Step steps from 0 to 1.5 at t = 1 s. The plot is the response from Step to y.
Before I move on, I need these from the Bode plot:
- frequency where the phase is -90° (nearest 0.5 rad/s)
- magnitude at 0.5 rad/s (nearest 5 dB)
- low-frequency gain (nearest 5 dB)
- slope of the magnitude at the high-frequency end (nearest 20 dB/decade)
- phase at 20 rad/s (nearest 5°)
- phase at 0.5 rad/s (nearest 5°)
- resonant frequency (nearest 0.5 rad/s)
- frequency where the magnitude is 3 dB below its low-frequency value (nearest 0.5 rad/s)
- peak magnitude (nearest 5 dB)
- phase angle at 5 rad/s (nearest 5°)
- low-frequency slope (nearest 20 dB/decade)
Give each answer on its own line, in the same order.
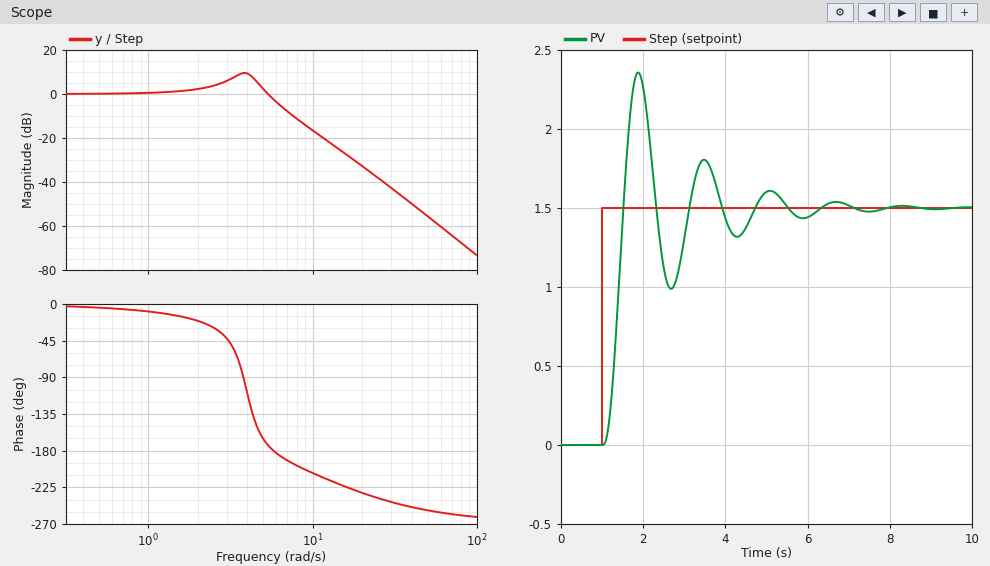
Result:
4.0 rad/s
0 dB
0 dB
-60 dB/decade
-230°
-5°
4.0 rad/s
6.0 rad/s
10 dB
-165°
0 dB/decade
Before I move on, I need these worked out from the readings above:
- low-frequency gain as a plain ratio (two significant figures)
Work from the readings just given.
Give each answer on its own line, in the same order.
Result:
1.0
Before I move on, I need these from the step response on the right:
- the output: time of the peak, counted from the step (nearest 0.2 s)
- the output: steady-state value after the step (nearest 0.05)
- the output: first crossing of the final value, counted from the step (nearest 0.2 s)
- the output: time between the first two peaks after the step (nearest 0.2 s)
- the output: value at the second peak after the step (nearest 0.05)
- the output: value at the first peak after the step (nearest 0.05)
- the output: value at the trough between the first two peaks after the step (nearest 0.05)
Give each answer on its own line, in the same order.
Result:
0.8 s
1.50
0.6 s
1.6 s
1.80
2.35
1.00
